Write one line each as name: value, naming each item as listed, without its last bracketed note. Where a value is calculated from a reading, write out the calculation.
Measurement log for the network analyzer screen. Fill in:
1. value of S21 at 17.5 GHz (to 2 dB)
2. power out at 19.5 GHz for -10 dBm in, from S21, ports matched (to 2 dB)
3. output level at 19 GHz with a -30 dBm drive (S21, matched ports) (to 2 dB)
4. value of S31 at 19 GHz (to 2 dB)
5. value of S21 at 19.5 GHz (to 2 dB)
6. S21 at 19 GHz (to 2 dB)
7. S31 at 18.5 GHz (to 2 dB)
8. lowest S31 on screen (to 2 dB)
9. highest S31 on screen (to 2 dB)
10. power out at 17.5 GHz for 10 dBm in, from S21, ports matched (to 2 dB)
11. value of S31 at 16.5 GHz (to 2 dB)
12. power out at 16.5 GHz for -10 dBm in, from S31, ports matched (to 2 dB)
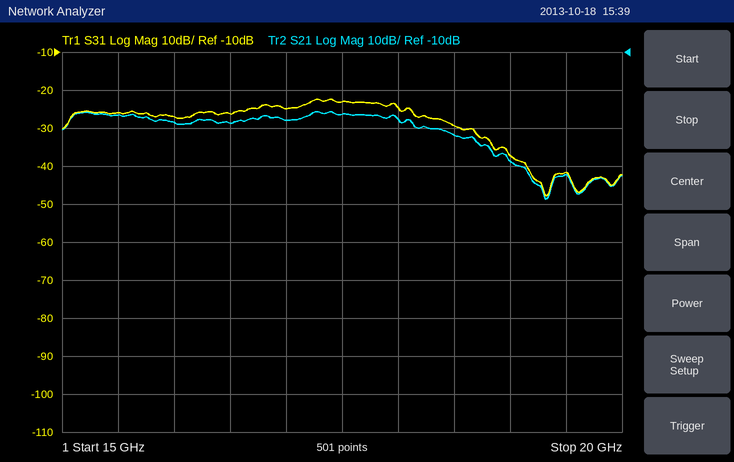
value of S21 at 17.5 GHz: -26 dB
power out at 19.5 GHz for -10 dBm in, from S21, ports matched: -10 dBm + (-42 dB) = -52 dBm
output level at 19 GHz with a -30 dBm drive (S21, matched ports): -30 dBm + (-38 dB) = -68 dBm
value of S31 at 19 GHz: -38 dB
value of S21 at 19.5 GHz: -42 dB
S21 at 19 GHz: -38 dB
S31 at 18.5 GHz: -30 dB
lowest S31 on screen: -48 dB
highest S31 on screen: -22 dB
power out at 17.5 GHz for 10 dBm in, from S21, ports matched: 10 dBm + (-26 dB) = -16 dBm
value of S31 at 16.5 GHz: -26 dB
power out at 16.5 GHz for -10 dBm in, from S31, ports matched: -10 dBm + (-26 dB) = -36 dBm
